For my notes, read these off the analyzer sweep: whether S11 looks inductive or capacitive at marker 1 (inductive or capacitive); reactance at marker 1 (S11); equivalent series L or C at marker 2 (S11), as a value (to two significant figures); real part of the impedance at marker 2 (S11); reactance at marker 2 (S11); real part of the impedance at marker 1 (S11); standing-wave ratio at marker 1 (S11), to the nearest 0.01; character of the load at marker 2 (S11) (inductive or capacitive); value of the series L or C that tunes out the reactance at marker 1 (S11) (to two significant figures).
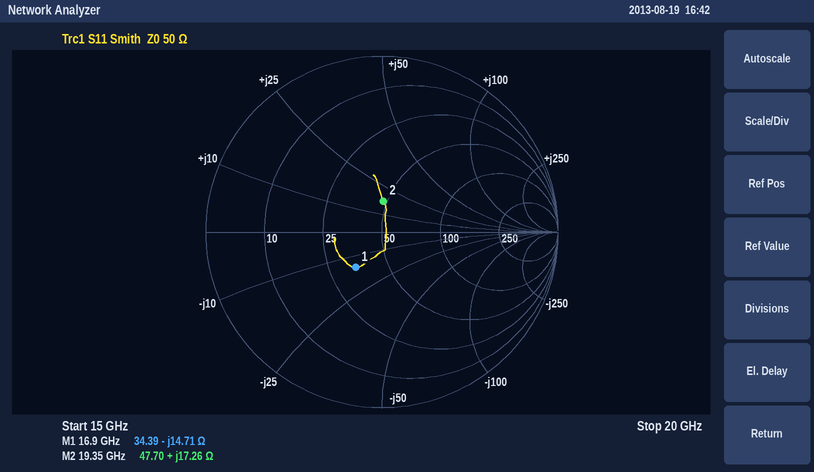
capacitive
-14.71 Ω
140 pH
47.70 Ω
+17.26 Ω
34.39 Ω
1.67
inductive
140 pH
